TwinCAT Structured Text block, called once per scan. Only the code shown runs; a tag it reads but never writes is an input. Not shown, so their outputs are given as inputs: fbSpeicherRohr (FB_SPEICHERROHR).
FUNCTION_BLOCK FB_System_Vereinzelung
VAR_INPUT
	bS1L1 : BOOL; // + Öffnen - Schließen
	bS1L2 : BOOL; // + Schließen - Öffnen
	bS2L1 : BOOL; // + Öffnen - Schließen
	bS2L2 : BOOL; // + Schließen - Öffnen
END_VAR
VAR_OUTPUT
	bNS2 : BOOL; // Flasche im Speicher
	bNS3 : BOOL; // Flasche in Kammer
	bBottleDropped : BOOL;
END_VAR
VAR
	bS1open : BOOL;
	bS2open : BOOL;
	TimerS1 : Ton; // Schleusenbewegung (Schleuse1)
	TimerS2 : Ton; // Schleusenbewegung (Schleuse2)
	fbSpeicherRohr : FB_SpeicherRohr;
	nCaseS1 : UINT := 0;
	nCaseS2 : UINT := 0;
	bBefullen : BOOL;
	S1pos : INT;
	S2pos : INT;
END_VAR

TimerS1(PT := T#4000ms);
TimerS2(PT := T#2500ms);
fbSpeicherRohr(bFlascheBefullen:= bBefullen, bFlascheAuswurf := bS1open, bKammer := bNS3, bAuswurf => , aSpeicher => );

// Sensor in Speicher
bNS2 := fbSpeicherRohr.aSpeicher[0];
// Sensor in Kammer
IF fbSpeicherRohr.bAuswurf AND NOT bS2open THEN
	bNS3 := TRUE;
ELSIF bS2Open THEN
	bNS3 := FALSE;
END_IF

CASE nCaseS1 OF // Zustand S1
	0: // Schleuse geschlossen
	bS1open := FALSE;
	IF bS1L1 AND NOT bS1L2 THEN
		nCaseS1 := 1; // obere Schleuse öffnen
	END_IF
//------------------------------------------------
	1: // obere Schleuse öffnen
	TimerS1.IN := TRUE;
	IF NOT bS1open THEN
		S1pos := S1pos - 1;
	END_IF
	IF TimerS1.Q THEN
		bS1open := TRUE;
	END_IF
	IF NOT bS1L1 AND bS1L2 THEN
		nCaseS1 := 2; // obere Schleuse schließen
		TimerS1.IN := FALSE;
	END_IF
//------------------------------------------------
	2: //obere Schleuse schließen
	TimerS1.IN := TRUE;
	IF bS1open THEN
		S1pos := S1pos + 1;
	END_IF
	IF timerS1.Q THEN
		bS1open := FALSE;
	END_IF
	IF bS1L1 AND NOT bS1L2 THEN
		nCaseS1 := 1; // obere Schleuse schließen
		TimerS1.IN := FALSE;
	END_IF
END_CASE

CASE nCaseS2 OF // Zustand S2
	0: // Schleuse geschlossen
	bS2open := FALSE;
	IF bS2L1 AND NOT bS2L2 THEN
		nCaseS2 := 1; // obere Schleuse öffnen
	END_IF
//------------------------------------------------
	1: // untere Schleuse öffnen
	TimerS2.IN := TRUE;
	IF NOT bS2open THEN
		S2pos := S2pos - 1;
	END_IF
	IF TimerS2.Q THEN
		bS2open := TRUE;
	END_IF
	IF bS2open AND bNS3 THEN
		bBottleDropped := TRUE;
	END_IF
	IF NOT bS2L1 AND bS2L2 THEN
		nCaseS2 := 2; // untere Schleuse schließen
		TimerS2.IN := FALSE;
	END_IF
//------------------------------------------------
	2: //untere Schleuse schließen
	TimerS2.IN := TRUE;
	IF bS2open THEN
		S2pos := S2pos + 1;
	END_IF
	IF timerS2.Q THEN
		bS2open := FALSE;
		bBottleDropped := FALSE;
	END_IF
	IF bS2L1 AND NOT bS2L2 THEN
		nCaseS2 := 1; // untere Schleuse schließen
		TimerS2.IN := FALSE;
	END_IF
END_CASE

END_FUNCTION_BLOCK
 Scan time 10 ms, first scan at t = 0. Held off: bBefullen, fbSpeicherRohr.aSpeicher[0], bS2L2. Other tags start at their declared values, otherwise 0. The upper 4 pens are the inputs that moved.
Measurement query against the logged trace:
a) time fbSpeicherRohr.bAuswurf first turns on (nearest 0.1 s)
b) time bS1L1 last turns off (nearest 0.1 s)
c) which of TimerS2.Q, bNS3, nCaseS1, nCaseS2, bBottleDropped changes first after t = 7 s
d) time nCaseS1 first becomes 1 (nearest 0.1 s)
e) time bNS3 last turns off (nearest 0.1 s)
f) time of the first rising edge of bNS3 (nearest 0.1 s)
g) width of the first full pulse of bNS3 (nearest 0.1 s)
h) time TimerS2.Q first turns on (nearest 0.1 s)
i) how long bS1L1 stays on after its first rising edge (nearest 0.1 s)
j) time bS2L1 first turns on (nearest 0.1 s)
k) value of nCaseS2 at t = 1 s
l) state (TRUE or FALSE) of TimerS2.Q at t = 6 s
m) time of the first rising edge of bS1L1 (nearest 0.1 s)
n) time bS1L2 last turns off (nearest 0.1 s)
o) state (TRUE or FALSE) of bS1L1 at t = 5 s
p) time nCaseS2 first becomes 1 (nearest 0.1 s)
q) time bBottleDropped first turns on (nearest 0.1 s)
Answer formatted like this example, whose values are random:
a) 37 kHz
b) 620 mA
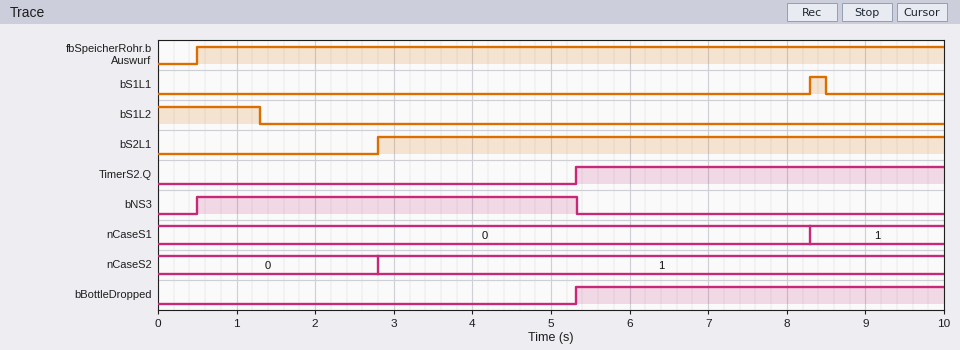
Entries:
a) 0.5 s
b) 8.5 s
c) nCaseS1
d) 8.3 s
e) 5.3 s
f) 0.5 s
g) 4.8 s
h) 5.3 s
i) 0.2 s
j) 2.8 s
k) 0
l) TRUE
m) 8.3 s
n) 1.3 s
o) FALSE
p) 2.8 s
q) 5.3 s
